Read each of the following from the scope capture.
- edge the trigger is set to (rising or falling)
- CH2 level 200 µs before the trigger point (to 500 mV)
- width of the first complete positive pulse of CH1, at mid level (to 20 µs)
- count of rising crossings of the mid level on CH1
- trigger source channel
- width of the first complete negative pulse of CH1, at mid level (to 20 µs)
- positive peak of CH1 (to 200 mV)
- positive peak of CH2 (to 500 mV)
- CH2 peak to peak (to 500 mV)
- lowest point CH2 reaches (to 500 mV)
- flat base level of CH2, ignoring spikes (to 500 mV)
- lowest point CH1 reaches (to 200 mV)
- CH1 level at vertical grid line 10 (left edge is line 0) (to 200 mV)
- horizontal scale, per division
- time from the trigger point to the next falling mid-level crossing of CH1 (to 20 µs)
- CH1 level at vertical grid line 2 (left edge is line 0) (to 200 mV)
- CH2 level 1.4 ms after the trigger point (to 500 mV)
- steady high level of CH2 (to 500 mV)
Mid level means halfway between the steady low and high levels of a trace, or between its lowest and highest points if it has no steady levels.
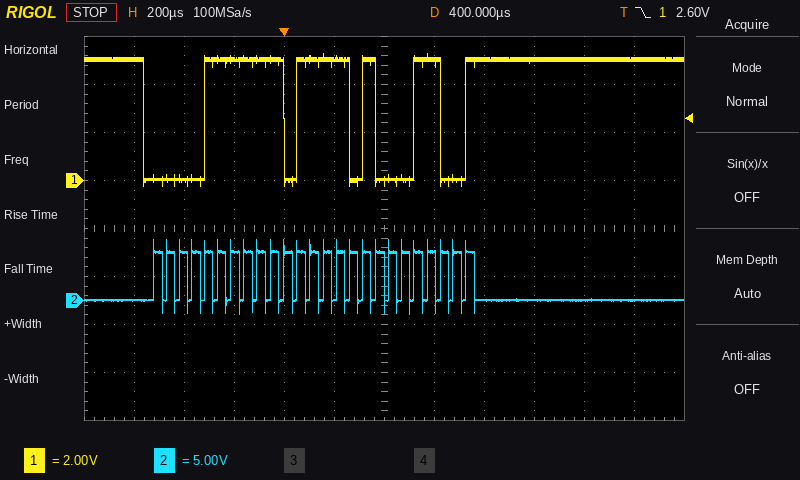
falling
5.0 V
320 µs
5
CH1
240 µs
5.2 V
6.5 V
8.0 V
-1.5 V
0.0 V
-200 mV
5.0 V
200 µs
260 µs
0.0 V
0.0 V
5.0 V
